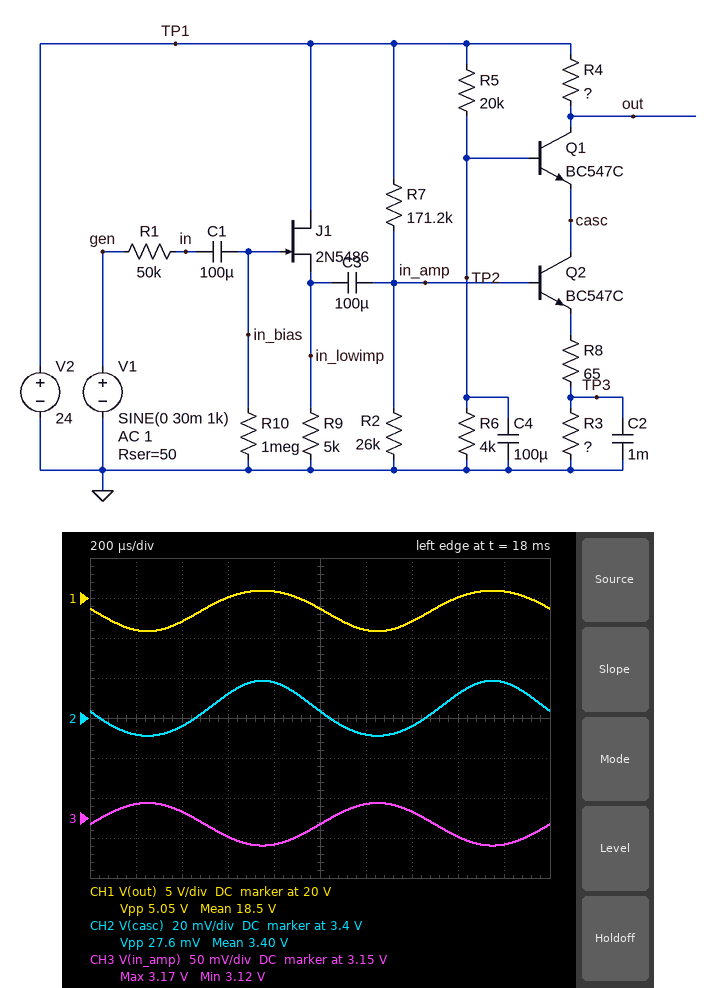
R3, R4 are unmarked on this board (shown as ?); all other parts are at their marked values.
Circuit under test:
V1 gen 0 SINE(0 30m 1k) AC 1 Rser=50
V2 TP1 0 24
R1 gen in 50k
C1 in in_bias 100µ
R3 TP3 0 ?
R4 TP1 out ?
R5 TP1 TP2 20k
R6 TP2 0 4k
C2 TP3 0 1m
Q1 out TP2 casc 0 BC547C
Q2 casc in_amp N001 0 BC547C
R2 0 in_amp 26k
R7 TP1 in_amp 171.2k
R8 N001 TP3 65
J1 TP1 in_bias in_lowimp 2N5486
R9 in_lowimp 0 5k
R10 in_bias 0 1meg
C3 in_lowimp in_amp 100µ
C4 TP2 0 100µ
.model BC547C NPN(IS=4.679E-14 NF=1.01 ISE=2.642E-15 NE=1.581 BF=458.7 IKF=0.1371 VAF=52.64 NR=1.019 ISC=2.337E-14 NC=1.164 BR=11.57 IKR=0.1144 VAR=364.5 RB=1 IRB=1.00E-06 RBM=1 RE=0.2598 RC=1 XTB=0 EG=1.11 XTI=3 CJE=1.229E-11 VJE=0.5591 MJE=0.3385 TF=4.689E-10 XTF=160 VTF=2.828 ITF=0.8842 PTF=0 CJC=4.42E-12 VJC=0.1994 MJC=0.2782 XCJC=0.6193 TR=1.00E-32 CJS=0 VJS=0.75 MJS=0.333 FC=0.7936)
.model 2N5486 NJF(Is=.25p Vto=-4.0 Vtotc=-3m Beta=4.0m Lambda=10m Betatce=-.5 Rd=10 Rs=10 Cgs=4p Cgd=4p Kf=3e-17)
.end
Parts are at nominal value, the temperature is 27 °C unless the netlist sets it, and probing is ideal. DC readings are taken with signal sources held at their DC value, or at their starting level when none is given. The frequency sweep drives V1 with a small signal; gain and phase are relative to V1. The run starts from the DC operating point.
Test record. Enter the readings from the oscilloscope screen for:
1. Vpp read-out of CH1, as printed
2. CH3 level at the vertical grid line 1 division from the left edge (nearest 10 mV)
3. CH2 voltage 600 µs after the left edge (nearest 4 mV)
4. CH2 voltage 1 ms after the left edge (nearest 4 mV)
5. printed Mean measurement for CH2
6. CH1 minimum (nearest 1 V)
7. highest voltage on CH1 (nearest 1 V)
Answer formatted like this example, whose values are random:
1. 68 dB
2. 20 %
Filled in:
1. 5.05 V
2. 3.17 V
3. 3.412 V
4. 3.404 V
5. 3.40 V
6. 16 V
7. 21 V
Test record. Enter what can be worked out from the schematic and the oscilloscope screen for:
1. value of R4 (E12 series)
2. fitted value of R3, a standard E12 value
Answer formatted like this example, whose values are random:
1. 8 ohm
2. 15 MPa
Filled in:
1. 12 kΩ
2. 5.6 kΩ
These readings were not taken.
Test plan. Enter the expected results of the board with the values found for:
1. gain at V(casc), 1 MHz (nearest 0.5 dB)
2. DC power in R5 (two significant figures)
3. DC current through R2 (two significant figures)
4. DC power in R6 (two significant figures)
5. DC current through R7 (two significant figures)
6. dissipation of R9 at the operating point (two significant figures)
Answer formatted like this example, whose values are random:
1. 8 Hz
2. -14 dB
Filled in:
1. -7.0 dB
2. 20 mW
3. 120 µA
4. 4.0 mW
5. 120 µA
6. 2.6 mW
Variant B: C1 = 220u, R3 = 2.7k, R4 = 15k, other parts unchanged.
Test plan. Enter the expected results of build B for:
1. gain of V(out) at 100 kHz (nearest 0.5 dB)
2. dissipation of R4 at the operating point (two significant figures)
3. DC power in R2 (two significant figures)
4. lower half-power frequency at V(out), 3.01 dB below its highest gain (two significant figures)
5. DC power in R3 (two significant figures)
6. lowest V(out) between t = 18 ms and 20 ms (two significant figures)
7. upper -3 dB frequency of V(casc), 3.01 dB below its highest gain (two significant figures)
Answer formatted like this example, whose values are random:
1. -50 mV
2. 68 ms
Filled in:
1. 43.0 dB
2. 12 mW
3. 370 µW
4. 1.8 Hz
5. 2.2 mW
6. 6.1 V
7. 3.8 MHz
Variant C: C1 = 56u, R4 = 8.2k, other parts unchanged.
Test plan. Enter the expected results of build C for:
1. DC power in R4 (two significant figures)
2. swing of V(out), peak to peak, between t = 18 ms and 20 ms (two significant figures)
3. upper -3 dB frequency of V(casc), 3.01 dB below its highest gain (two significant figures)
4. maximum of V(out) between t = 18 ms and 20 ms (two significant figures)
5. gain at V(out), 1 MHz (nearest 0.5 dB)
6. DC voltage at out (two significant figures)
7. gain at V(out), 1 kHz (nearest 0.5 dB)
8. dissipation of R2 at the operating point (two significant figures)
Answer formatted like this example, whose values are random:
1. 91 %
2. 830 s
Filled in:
1. 1.6 mW
2. 3.5 V
3. 4.1 MHz
4. 22 V
5. 35.0 dB
6. 20 V
7. 35.5 dB
8. 380 µW
